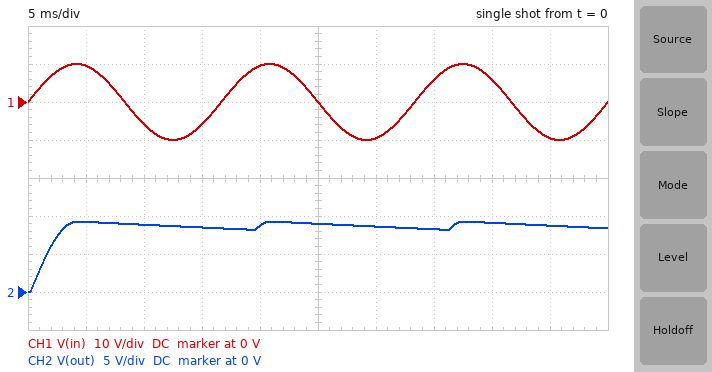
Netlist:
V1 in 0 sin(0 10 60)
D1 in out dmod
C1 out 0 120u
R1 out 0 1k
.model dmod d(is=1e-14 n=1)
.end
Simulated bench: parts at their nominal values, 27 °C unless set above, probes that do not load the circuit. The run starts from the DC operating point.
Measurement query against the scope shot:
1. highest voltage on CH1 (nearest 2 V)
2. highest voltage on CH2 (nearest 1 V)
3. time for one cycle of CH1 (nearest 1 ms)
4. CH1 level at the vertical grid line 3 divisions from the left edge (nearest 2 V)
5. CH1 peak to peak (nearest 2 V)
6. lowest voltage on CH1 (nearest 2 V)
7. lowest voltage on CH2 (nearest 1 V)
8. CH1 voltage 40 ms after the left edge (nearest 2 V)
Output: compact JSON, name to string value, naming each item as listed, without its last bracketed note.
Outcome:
{"highest voltage on CH1": "10 V", "highest voltage on CH2": "9 V", "time for one cycle of CH1": "17 ms", "CH1 level at the vertical grid line 3 divisions from the left edge": "-6 V", "CH1 peak to peak": "20 V", "lowest voltage on CH1": "-10 V", "lowest voltage on CH2": "0 V", "CH1 voltage 40 ms after the left edge": "6 V"}
